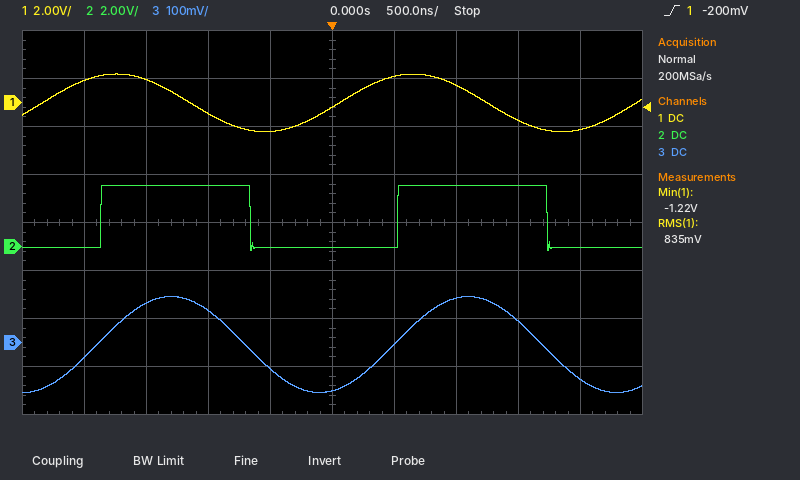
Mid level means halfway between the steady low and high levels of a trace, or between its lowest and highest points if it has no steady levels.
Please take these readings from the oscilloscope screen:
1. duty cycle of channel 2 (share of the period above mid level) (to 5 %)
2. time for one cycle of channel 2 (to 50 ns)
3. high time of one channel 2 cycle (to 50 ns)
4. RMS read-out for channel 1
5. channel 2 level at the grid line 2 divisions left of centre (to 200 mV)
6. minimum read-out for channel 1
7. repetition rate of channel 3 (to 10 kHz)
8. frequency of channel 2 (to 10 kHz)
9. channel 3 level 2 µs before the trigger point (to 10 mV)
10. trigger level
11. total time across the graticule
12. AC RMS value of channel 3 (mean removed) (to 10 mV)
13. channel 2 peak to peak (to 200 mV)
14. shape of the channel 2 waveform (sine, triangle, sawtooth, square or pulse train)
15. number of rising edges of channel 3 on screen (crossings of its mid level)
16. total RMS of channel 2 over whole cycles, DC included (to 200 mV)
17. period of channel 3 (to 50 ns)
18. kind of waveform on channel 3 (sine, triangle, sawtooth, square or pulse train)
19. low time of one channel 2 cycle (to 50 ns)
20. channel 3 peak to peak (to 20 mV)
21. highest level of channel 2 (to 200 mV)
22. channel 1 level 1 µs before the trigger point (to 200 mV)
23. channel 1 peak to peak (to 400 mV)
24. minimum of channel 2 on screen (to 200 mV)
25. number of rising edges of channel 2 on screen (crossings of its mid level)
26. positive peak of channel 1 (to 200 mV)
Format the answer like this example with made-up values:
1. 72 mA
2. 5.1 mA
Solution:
1. 50 %
2. 2.40 µs
3. 1.20 µs
4. 835 mV
5. 2.6 V
6. -1.22 V
7. 420 kHz
8. 420 kHz
9. -30 mV
10. -200 mV
11. 5 µs
12. 70 mV
13. 2.8 V
14. square
15. 2
16. 1.8 V
17. 2.40 µs
18. sine
19. 1.20 µs
20. 200 mV
21. 2.6 V
22. -400 mV
23. 2.4 V
24. -200 mV
25. 2
26. 1.2 V
